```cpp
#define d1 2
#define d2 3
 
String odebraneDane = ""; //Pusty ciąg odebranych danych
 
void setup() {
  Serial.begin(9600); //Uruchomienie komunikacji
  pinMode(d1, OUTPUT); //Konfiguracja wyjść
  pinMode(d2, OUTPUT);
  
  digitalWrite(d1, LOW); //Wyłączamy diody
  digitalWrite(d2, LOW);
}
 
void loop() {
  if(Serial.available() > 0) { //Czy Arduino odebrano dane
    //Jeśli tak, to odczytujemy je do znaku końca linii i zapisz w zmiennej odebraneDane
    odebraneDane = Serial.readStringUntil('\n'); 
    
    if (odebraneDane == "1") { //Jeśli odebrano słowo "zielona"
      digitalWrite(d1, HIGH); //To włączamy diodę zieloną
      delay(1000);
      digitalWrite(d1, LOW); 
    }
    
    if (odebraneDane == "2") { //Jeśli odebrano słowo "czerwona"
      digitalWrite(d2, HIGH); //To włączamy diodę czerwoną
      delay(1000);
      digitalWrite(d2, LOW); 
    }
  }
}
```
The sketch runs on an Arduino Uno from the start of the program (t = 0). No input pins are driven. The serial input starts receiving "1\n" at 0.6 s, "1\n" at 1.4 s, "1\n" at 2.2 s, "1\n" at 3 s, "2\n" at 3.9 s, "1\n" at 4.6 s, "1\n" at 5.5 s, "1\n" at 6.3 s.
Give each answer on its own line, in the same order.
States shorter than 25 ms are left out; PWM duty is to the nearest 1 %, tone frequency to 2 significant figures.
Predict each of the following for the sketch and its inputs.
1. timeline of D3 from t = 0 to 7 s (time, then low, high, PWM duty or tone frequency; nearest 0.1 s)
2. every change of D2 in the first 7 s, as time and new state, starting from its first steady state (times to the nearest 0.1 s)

0 s low; 4.6 s high; 5.6 s low
0 s low; 0.6 s high; 4.6 s low; 5.6 s high
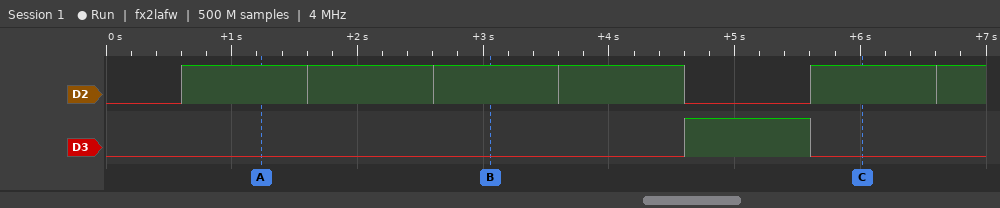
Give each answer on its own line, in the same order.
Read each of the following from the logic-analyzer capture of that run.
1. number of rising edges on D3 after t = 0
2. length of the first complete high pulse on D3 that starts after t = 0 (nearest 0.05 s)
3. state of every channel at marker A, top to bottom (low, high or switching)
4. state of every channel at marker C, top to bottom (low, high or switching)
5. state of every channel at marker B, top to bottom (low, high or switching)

1
1.00 s
D2 high, D3 low
D2 high, D3 low
D2 high, D3 low
